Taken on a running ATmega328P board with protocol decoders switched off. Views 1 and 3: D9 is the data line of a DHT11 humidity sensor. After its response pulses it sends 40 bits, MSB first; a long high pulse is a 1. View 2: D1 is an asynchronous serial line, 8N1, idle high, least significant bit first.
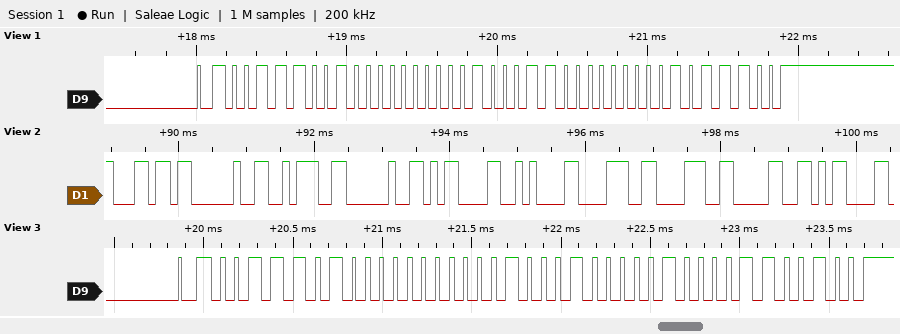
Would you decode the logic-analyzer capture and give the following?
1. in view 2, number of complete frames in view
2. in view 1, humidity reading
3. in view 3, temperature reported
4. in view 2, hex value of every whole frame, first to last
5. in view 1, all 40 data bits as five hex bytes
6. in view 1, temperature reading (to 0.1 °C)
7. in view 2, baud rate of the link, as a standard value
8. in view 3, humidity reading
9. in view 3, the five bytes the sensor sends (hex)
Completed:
10
57 %
34.8 °C
0x6C 0x20 0x3A 0x20 0x0D 0x0A 0x38 0x38 0x30 0x0D
39 00 23 00 5C
35.0 °C
9600 baud
58 %
3A 00 22 08 64
